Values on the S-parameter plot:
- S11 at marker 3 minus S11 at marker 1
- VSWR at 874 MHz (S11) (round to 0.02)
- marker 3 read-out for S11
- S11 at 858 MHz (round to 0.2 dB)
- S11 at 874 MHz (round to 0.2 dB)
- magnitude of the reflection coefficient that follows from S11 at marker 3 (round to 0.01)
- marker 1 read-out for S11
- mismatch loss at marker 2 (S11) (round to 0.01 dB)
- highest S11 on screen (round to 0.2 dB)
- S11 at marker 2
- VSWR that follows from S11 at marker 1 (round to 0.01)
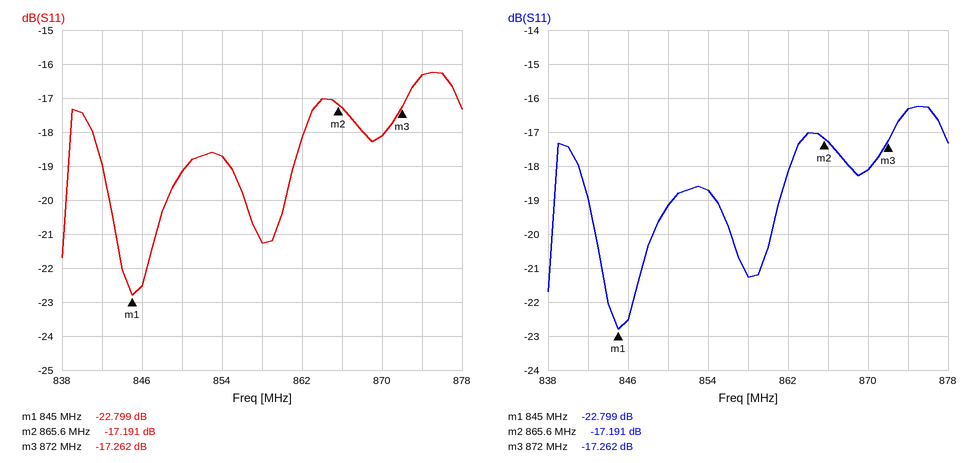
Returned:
5.537 dB
1.36
-17.262 dB
-21.2 dB
-16.4 dB
0.14
-22.799 dB
0.08 dB
-16.2 dB
-17.191 dB
1.16
